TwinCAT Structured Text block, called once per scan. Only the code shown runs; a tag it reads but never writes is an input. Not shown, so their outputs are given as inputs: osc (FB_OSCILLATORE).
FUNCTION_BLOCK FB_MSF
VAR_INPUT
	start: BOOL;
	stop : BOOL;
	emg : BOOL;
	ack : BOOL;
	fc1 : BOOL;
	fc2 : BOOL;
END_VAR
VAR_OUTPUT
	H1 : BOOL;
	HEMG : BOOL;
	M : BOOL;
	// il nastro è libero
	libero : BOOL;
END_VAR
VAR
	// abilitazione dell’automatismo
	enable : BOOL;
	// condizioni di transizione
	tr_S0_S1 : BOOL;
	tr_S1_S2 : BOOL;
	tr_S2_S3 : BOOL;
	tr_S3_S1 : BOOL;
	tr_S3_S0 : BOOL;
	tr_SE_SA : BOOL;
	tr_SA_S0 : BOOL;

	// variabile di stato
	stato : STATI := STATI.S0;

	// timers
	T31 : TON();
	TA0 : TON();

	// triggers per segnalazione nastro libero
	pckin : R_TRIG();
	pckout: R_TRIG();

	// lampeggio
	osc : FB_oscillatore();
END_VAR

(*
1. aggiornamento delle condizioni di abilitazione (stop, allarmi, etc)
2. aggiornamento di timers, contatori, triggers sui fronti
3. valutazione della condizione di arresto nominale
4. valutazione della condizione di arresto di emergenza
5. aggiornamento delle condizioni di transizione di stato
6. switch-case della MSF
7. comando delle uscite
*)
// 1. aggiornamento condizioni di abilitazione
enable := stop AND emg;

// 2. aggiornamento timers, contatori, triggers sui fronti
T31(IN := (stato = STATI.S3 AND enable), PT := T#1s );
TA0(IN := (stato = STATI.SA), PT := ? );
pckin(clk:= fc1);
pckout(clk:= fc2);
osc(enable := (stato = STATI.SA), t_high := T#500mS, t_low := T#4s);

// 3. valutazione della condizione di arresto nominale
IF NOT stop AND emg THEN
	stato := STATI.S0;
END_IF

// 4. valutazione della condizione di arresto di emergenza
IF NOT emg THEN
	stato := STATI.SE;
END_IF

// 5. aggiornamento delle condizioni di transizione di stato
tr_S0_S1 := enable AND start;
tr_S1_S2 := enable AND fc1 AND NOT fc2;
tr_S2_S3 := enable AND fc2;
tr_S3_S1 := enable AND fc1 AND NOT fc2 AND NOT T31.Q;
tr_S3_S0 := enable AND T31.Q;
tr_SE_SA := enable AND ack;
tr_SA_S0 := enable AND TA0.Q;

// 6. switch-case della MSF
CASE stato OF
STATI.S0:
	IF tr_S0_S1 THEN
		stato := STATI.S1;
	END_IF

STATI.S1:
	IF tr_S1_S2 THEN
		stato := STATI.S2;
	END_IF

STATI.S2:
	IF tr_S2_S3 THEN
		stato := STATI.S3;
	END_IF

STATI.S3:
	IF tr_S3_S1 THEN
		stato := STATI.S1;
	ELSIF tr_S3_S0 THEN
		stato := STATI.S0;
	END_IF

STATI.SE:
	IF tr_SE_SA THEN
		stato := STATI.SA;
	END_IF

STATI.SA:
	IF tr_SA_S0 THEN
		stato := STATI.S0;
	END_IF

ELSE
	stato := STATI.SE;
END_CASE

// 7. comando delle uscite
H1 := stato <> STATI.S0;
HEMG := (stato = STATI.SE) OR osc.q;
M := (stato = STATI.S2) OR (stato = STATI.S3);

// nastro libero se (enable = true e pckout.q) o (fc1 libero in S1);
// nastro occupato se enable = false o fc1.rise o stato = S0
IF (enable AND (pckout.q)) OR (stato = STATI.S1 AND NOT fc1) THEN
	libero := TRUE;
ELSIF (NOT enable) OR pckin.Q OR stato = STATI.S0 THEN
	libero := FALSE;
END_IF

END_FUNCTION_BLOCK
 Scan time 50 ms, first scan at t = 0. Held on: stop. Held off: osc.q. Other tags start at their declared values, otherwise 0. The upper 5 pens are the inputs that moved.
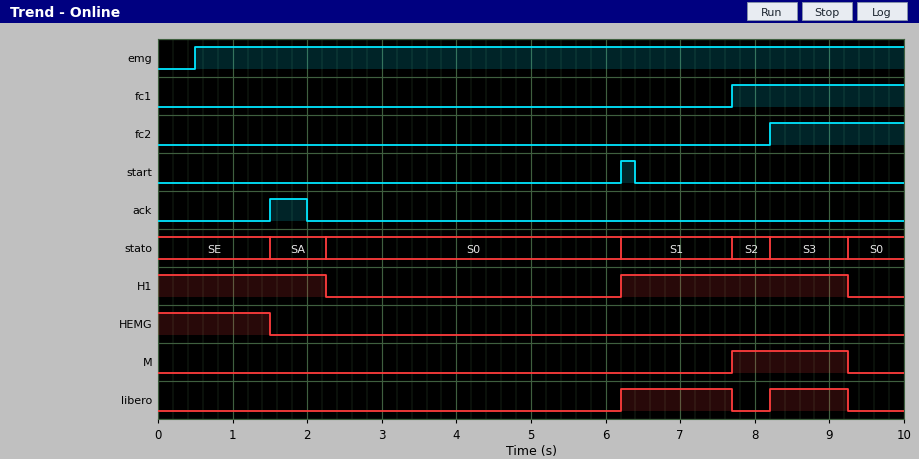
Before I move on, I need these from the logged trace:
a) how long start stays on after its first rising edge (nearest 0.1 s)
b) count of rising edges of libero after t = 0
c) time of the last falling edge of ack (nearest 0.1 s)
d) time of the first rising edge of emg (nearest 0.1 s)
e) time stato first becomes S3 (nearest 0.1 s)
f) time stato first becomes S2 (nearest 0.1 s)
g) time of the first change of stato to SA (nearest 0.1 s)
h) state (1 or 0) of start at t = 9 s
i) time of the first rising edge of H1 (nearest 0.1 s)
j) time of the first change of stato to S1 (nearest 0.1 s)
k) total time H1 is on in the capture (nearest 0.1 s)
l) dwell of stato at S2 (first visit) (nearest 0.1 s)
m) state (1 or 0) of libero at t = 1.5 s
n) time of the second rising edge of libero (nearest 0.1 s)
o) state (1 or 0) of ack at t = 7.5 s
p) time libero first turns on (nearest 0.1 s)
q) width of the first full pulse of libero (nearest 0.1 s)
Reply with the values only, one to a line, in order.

0.2 s
2
2.0 s
0.5 s
8.2 s
7.7 s
1.5 s
0
6.2 s
6.2 s
5.3 s
0.5 s
0
8.2 s
0
6.2 s
1.5 s
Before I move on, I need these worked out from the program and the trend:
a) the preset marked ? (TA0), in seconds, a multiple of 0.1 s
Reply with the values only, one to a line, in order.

0.7 s
